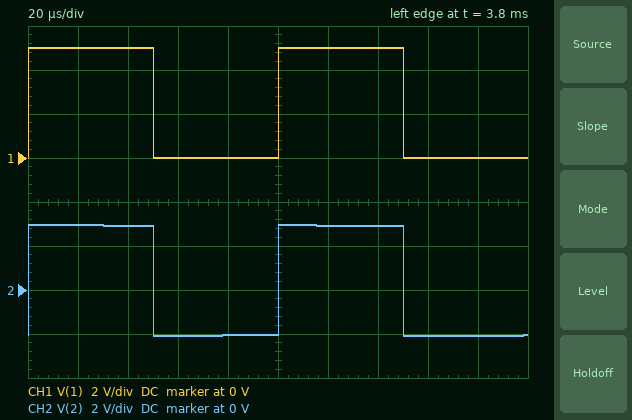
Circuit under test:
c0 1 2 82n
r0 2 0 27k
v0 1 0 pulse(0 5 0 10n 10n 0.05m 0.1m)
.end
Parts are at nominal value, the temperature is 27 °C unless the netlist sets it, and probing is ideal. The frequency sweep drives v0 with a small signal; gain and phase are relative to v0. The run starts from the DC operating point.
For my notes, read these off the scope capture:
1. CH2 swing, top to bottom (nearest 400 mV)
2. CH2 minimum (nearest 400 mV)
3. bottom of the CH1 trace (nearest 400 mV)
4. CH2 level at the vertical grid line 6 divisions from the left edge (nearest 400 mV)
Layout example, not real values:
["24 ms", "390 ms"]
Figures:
["5.2 V", "-2.0 V", "0 V", "2.8 V"]
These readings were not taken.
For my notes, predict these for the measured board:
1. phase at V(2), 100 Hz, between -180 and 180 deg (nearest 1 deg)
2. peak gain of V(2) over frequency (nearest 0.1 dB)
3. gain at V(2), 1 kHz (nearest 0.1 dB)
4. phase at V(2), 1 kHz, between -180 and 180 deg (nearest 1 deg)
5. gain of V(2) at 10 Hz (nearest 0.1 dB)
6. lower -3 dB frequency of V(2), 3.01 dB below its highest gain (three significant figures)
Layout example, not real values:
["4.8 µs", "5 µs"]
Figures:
["36 deg", "0 dB", "0 dB", "4 deg", "-17.2 dB", "71.9 Hz"]
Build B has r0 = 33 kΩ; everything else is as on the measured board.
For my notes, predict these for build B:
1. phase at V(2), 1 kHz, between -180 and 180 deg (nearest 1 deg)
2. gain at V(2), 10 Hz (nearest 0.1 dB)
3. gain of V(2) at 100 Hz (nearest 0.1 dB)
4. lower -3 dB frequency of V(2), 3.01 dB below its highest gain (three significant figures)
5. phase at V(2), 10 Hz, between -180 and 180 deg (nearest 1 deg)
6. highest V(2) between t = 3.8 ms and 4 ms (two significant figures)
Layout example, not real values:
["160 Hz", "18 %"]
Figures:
["3 deg", "-15.5 dB", "-1.3 dB", "58.8 Hz", "80 deg", "3.1 V"]
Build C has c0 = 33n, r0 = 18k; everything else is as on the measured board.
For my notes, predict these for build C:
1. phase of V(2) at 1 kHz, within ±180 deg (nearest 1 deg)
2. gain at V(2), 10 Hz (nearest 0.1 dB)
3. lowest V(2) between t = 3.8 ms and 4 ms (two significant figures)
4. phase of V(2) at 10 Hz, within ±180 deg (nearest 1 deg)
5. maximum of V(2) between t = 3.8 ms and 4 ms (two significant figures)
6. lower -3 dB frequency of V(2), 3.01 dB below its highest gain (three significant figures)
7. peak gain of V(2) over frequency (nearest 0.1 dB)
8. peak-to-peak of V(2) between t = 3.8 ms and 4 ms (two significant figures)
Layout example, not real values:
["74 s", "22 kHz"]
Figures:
["15 deg", "-28.6 dB", "-2.6 V", "88 deg", "2.6 V", "268 Hz", "0 dB", "5.2 V"]
